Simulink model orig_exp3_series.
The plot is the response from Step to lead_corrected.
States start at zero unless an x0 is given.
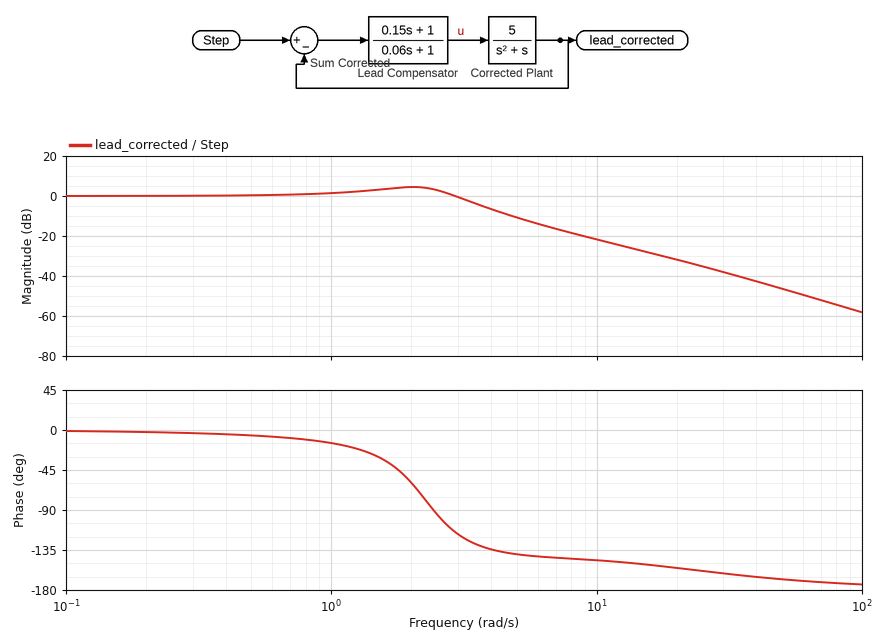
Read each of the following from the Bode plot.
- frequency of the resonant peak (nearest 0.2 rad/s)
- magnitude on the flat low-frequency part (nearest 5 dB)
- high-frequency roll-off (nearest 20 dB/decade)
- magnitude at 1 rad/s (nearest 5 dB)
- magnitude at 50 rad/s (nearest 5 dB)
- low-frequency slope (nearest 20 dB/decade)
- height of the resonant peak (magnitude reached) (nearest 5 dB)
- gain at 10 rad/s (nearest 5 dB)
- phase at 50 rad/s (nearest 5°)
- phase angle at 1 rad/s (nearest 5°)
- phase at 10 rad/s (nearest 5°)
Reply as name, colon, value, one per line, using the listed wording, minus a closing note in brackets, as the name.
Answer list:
frequency of the resonant peak: 2.0 rad/s
magnitude on the flat low-frequency part: 0 dB
high-frequency roll-off: -40 dB/decade
magnitude at 1 rad/s: 0 dB
magnitude at 50 rad/s: -45 dB
low-frequency slope: 0 dB/decade
height of the resonant peak (magnitude reached): 5 dB
gain at 10 rad/s: -20 dB
phase at 50 rad/s: -170°
phase angle at 1 rad/s: -15°
phase at 10 rad/s: -145°
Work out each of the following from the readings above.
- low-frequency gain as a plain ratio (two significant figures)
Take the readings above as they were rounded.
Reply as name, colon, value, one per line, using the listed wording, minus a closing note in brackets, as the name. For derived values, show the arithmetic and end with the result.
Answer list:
low-frequency gain as a plain ratio: 10^(0 / 20) = 1.0
